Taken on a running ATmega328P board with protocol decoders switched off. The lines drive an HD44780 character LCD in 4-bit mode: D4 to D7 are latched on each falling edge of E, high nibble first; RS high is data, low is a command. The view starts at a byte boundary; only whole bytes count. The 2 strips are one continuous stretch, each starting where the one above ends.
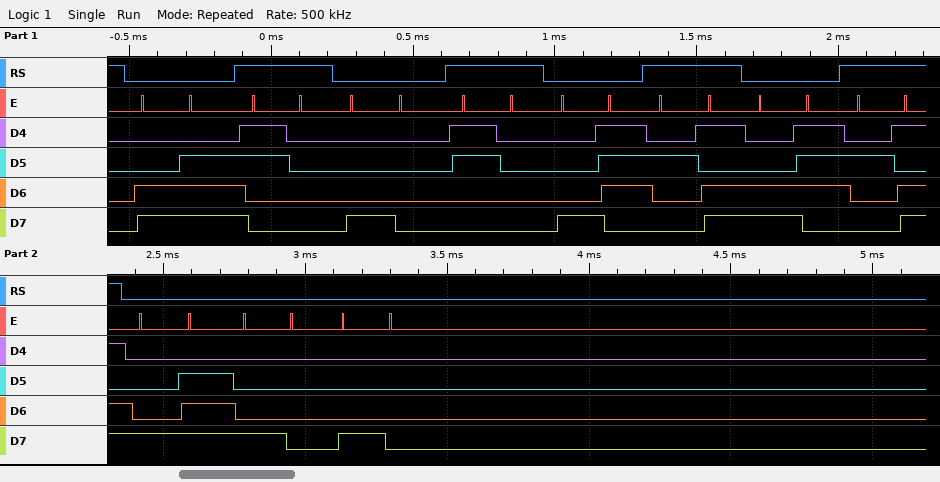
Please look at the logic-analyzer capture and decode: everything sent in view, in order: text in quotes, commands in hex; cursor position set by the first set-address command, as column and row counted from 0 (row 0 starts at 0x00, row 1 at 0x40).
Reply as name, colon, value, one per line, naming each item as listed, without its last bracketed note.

everything sent in view, in order: text in quotes, commands in hex: 0xCE "0" 0x80 "0" 0x87 "-" 0xC7 "-" 0x8E 0x80 0x80
cursor position set by the first set-address command, as column and row counted from 0: column 14, row 1
